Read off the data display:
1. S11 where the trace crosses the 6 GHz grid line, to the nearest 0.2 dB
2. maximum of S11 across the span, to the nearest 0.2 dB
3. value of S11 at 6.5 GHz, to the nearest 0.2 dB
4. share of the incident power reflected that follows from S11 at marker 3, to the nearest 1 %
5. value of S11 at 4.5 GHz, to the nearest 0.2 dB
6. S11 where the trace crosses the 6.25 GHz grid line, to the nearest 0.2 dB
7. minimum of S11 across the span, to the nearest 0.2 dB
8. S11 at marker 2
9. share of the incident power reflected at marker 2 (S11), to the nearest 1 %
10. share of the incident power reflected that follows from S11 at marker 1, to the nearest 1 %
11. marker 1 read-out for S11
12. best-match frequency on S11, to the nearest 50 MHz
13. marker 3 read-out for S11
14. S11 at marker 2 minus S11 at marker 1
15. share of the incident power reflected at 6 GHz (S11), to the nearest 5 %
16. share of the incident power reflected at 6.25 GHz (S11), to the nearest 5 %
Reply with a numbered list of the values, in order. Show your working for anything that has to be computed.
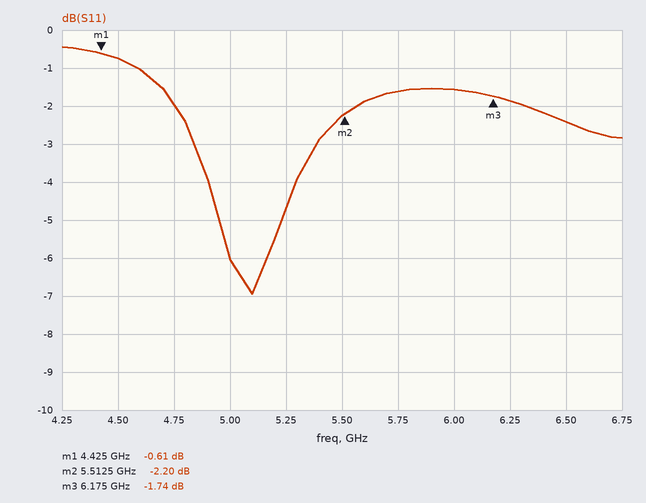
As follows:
1. -1.6 dB
2. -0.4 dB
3. -2.4 dB
4. 10^(-1.74/10) ≈ 67 %
5. -0.8 dB
6. -1.8 dB
7. -7.0 dB
8. -2.20 dB
9. 10^(-2.2/10) ≈ 60 %
10. 10^(-0.61/10) ≈ 87 %
11. -0.61 dB
12. 5.10 GHz
13. -1.74 dB
14. -2.2 − (-0.61) = -1.59 dB
15. 10^(-1.6/10) ≈ 69.2 %, so 70 % to the nearest 5 %
16. 10^(-1.8/10) ≈ 66.1 %, so 65 % to the nearest 5 %
